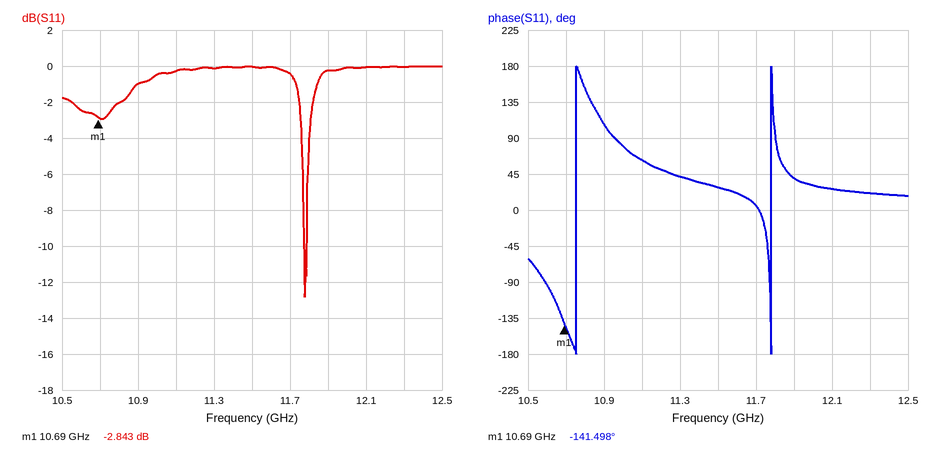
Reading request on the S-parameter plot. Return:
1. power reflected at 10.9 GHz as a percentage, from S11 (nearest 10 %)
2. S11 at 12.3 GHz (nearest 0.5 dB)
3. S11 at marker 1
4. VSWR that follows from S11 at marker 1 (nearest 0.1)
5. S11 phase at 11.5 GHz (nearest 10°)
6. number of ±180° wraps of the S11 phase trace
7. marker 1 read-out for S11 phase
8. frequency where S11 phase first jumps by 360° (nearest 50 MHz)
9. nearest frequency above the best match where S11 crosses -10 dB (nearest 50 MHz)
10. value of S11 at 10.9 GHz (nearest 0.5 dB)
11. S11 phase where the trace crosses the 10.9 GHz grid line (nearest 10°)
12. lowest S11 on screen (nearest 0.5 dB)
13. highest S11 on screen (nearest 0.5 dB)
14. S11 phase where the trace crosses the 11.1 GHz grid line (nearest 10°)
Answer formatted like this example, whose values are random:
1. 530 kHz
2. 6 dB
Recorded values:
1. 80 %
2. 0.0 dB
3. -2.843 dB
4. 6.2
5. 30°
6. 2
7. -141.498°
8. 10.75 GHz
9. 11.80 GHz
10. -1.0 dB
11. 110°
12. -13.0 dB
13. 0.0 dB
14. 60°
